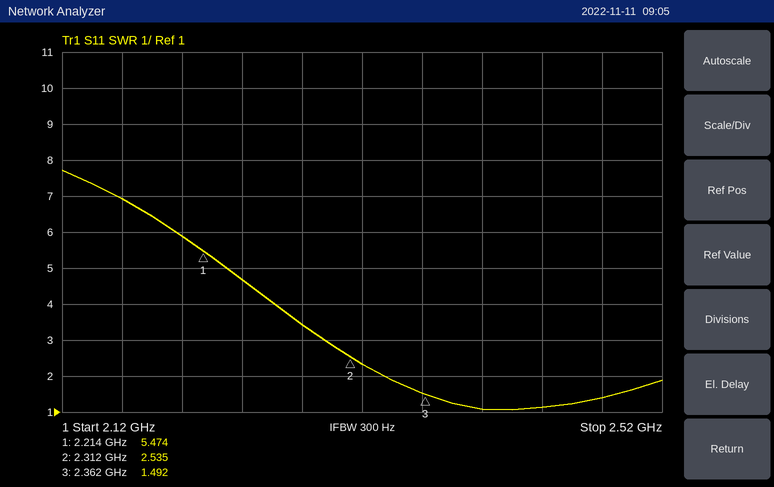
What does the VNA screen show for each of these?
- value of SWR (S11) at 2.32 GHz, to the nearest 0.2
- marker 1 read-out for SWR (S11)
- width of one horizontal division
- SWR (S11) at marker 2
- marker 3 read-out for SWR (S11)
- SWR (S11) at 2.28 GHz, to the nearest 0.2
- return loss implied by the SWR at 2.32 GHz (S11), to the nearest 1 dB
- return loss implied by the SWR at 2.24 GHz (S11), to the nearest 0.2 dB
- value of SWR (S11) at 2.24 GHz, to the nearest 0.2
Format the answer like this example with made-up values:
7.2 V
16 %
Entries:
2.4
5.474
40 MHz
2.535
1.492
3.4
8 dB
3.8 dB
4.6
